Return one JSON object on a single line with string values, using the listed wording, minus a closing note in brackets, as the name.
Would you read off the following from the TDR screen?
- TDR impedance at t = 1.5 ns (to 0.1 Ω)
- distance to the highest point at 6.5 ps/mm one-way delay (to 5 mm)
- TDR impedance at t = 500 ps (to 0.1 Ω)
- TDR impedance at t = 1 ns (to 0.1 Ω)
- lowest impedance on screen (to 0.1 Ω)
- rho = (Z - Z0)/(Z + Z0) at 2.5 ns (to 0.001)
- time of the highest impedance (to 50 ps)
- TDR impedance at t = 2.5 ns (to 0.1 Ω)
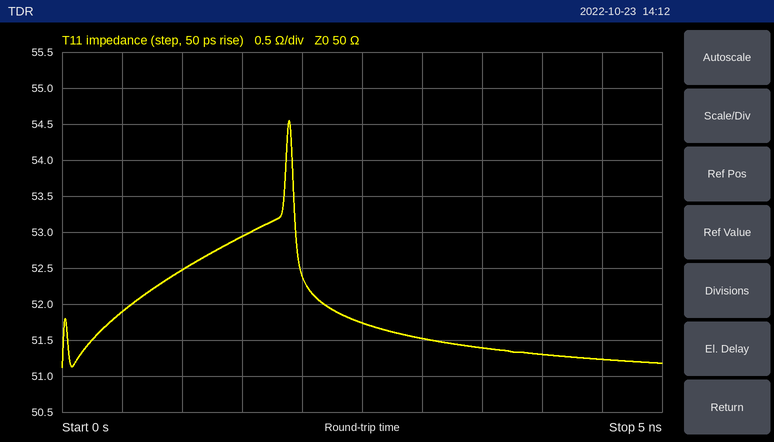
{"TDR impedance at t = 1.5 ns": "52.9 Ω", "distance to the highest point at 6.5 ps/mm one-way delay": "145 mm", "TDR impedance at t = 500 ps": "51.9 Ω", "TDR impedance at t = 1 ns": "52.5 Ω", "lowest impedance on screen": "51.1 Ω", "rho = (Z - Z0)/(Z + Z0) at 2.5 ns": "+0.017", "time of the highest impedance": "1.90 ns", "TDR impedance at t = 2.5 ns": "51.7 Ω"}
